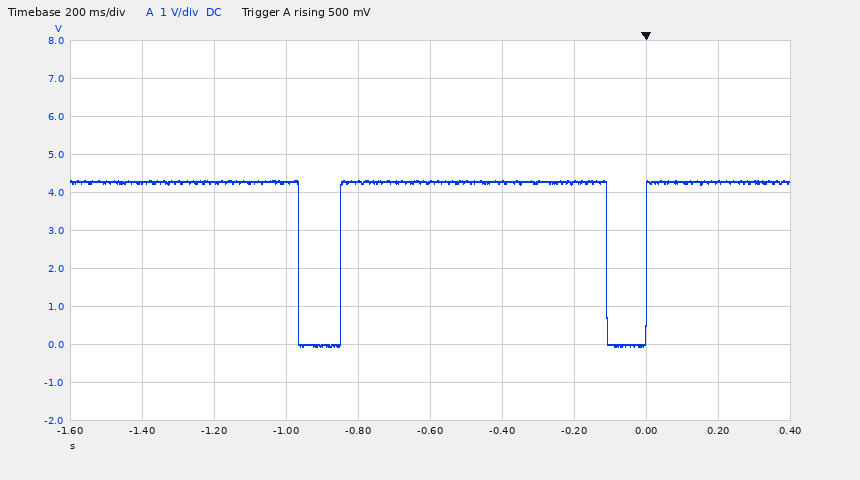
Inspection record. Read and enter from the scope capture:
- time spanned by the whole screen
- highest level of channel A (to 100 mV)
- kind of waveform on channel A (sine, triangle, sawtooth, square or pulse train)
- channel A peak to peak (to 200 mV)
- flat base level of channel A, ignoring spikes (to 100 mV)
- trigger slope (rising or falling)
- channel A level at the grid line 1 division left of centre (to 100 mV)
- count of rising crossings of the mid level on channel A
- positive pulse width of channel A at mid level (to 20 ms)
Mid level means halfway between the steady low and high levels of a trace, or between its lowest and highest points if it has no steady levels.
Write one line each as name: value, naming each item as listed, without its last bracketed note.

time spanned by the whole screen: 2 s
highest level of channel A: 4.3 V
kind of waveform on channel A: pulse train
channel A peak to peak: 4.4 V
flat base level of channel A, ignoring spikes: 0.0 V
trigger slope: rising
channel A level at the grid line 1 division left of centre: 4.3 V
count of rising crossings of the mid level on channel A: 2
positive pulse width of channel A at mid level: 740 ms
